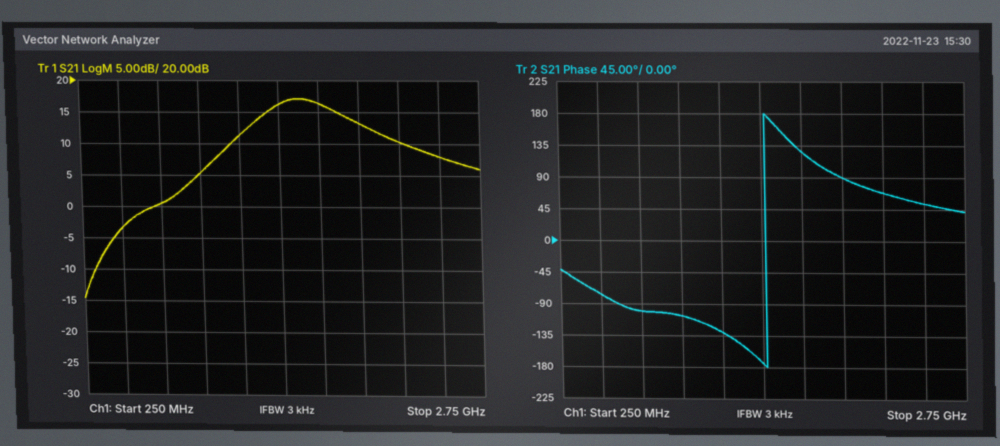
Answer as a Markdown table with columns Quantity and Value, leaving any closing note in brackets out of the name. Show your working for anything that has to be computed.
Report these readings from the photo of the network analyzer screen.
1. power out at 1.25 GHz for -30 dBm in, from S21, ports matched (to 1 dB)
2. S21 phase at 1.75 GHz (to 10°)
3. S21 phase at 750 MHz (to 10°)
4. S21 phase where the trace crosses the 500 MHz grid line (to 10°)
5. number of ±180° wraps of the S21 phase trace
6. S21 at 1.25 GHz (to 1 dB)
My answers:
| Quantity | Value |
|---|---|
| power out at 1.25 GHz for -30 dBm in, from S21, ports matched | -30 dBm + (11 dB) = -19 dBm |
| S21 phase at 1.75 GHz | 130° |
| S21 phase at 750 MHz | -100° |
| S21 phase where the trace crosses the 500 MHz grid line | -80° |
| number of ±180° wraps of the S21 phase trace | 1 |
| S21 at 1.25 GHz | 11 dB |
